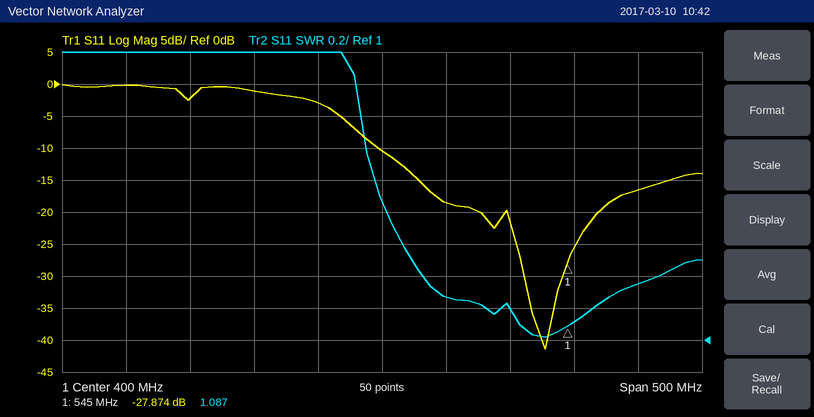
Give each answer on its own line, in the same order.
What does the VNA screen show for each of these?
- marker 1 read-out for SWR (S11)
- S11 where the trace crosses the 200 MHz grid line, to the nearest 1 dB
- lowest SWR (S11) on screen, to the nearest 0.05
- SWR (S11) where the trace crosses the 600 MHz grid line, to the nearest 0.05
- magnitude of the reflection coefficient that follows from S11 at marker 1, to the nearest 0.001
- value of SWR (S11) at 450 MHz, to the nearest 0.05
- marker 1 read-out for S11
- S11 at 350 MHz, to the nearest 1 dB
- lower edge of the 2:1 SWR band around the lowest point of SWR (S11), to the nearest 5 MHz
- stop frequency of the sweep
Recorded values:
1.087
0 dB
1.00
1.35
0.040
1.25
-27.874 dB
-3 dB
395 MHz
650 MHz
